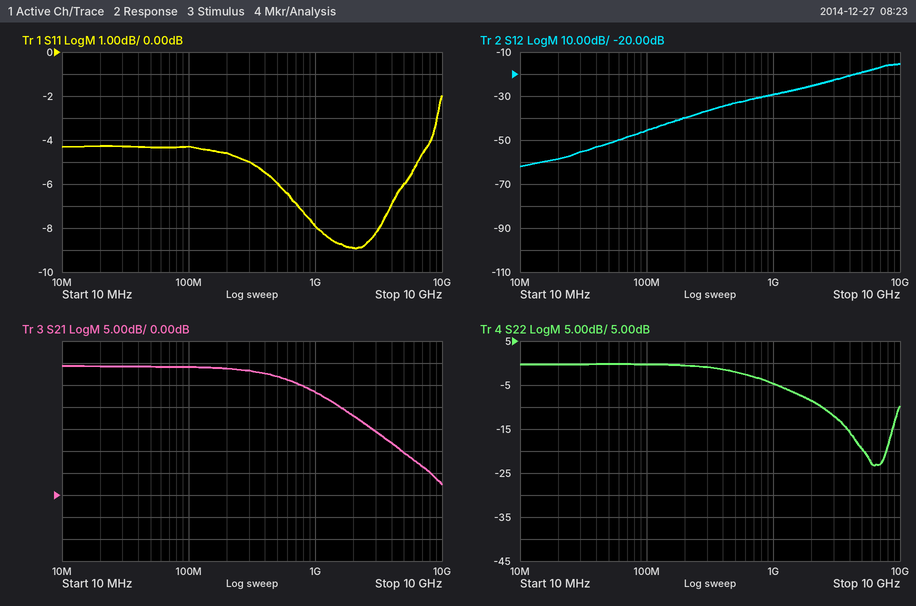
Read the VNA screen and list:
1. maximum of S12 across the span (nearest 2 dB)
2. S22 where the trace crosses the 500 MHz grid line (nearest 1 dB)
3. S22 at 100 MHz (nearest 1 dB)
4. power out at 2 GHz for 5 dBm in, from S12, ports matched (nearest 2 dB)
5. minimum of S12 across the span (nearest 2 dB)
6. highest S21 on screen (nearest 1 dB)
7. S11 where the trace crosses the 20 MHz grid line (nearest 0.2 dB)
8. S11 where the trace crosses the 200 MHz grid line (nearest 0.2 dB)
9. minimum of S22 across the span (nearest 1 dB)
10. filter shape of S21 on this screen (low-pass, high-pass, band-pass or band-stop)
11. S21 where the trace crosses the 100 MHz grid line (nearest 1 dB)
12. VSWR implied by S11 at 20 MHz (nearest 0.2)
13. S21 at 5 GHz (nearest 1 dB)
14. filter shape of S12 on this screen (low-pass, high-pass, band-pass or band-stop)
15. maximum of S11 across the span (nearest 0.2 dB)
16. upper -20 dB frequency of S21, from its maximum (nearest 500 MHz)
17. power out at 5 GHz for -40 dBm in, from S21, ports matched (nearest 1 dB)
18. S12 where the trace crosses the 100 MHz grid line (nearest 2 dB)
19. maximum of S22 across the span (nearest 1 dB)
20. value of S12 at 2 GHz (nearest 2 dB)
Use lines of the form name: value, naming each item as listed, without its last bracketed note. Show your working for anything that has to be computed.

maximum of S12 across the span: -16 dB
S22 where the trace crosses the 500 MHz grid line: -2 dB
S22 at 100 MHz: 0 dB
power out at 2 GHz for 5 dBm in, from S12, ports matched: 5 dBm + (-26 dB) = -20 dBm
minimum of S12 across the span: -62 dB
highest S21 on screen: 29 dB
S11 where the trace crosses the 20 MHz grid line: -4.2 dB
S11 where the trace crosses the 200 MHz grid line: -4.6 dB
minimum of S22 across the span: -23 dB
filter shape of S21 on this screen: low-pass
S21 where the trace crosses the 100 MHz grid line: 29 dB
VSWR implied by S11 at 20 MHz: |Γ| = 10^(-4.2/20) = 0.6166; VSWR = (1 + 0.6166)/(1 − 0.6166) ≈ 4.2
S21 at 5 GHz: 10 dB
filter shape of S12 on this screen: high-pass
maximum of S11 across the span: -2.0 dB
upper -20 dB frequency of S21, from its maximum: 5.0 GHz
power out at 5 GHz for -40 dBm in, from S21, ports matched: -40 dBm + (10 dB) = -30 dBm
S12 where the trace crosses the 100 MHz grid line: -46 dB
maximum of S22 across the span: 0 dB
value of S12 at 2 GHz: -26 dB
